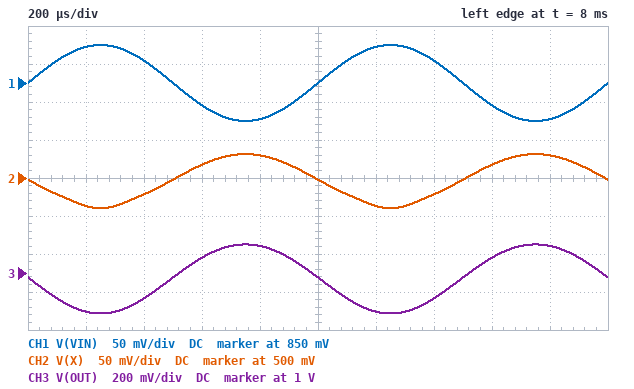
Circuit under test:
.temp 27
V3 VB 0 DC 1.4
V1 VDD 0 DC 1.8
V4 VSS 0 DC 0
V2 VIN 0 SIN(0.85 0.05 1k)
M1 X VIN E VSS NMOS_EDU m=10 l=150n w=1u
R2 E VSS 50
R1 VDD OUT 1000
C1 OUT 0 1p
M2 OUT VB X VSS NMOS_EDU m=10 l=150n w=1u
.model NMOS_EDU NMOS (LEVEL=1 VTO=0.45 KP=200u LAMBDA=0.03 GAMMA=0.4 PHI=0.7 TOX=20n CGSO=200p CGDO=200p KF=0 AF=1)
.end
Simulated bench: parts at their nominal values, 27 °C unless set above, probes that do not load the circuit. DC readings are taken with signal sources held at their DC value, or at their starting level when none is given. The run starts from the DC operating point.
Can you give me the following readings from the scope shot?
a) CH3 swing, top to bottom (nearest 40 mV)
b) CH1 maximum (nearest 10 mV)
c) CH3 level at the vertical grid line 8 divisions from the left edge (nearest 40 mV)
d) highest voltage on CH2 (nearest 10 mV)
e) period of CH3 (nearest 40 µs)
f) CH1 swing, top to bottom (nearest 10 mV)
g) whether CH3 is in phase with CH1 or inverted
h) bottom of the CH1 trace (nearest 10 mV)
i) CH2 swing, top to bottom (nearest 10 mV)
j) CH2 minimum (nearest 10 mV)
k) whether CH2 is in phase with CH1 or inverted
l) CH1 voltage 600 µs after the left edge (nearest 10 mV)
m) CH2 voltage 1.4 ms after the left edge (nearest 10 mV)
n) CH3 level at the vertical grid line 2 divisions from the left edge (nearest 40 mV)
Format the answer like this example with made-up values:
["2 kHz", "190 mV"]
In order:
["360 mV", "900 mV", "1.08 V", "530 mV", "1.00 ms", "100 mV", "inverted", "800 mV", "70 mV", "460 mV", "inverted", "820 mV", "480 mV", "880 mV"]
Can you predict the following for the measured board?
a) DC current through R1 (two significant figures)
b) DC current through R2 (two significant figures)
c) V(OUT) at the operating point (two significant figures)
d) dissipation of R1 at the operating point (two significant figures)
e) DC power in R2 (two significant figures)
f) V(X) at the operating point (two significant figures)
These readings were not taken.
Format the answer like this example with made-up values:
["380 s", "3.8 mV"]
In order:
["820 µA", "820 µA", "980 mV", "680 µW", "34 µW", "500 mV"]
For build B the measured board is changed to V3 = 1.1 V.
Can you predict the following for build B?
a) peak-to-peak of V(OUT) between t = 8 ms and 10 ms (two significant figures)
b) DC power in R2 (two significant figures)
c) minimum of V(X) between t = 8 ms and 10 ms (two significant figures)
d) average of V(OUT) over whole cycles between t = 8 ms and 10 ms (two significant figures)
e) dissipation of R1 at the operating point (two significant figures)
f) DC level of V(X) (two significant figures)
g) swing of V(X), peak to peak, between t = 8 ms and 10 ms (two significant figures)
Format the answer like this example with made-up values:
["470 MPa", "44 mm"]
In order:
["190 mV", "27 µW", "250 mV", "1.1 V", "540 µW", "260 mV", "37 mV"]
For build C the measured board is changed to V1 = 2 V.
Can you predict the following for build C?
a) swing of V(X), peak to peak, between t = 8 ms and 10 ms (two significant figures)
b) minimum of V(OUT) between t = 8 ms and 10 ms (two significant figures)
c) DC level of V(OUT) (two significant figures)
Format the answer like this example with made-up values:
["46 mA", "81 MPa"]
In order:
["66 mV", "990 mV", "1.2 V"]
